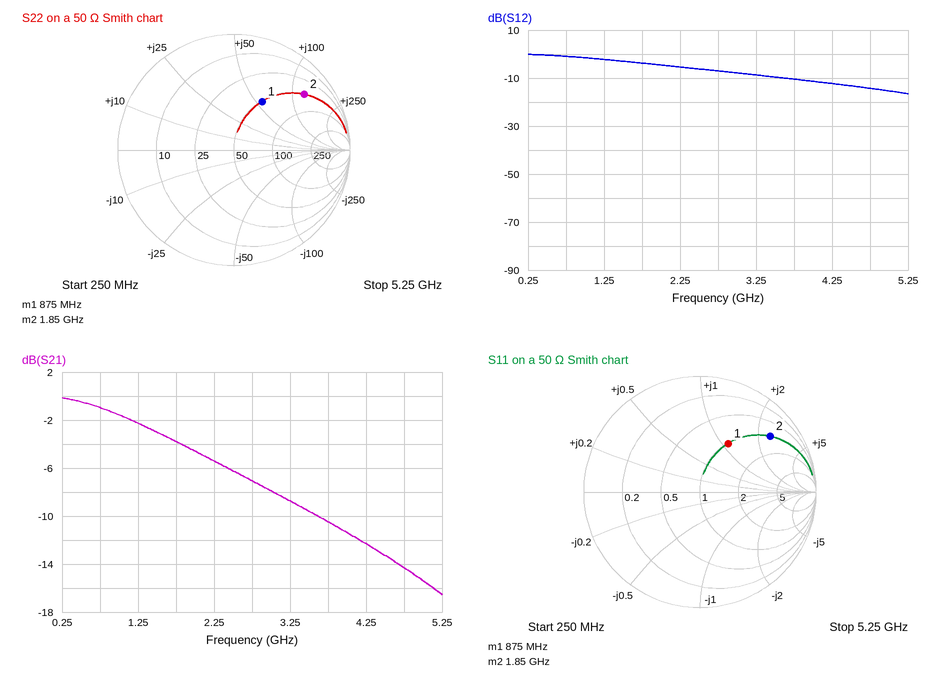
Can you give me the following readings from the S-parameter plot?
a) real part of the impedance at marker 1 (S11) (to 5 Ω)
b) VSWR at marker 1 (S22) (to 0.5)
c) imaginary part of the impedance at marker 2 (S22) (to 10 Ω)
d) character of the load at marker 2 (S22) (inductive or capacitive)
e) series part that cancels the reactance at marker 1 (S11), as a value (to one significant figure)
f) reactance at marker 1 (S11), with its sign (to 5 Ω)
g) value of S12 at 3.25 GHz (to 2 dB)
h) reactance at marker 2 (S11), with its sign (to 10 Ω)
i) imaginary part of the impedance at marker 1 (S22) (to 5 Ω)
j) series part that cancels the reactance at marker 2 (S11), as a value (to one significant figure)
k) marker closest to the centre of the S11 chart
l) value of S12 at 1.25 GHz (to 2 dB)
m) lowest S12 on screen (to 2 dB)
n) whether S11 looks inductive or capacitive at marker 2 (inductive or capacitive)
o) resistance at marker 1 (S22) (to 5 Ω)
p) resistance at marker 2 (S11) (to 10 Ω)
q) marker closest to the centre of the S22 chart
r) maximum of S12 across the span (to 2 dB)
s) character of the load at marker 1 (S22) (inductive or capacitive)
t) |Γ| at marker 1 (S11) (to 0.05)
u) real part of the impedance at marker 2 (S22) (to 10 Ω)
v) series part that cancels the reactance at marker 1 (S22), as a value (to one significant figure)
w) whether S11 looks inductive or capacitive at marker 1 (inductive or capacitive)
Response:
50 Ω
3.0
+120 Ω
inductive
3 pF
+55 Ω
-8 dB
+120 Ω
+55 Ω
700 fF
marker 1
-2 dB
-16 dB
inductive
50 Ω
50 Ω
marker 1
0 dB
inductive
0.50
50 Ω
3 pF
inductive
